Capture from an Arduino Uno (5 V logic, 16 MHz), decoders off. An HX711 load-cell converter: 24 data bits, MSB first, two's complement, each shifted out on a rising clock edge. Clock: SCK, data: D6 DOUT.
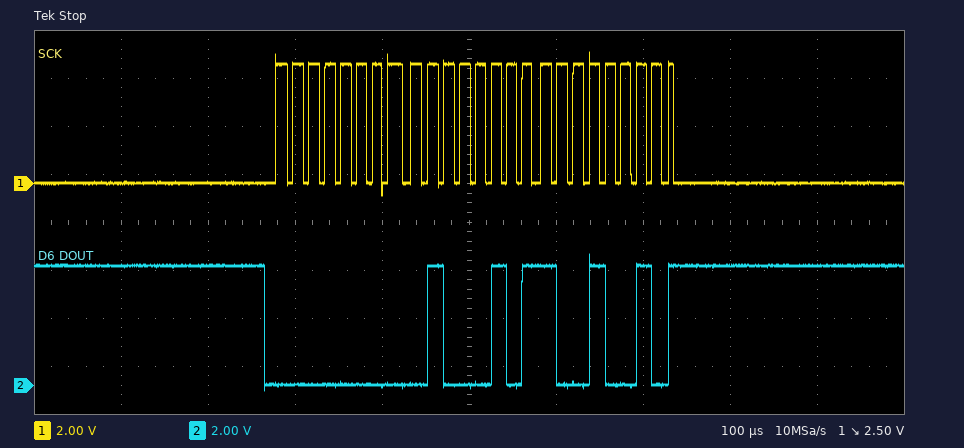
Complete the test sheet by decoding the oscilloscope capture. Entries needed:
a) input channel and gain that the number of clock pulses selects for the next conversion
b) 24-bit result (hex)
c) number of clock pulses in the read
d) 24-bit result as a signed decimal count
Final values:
channel A, gain 128
0x004592
25
17810
